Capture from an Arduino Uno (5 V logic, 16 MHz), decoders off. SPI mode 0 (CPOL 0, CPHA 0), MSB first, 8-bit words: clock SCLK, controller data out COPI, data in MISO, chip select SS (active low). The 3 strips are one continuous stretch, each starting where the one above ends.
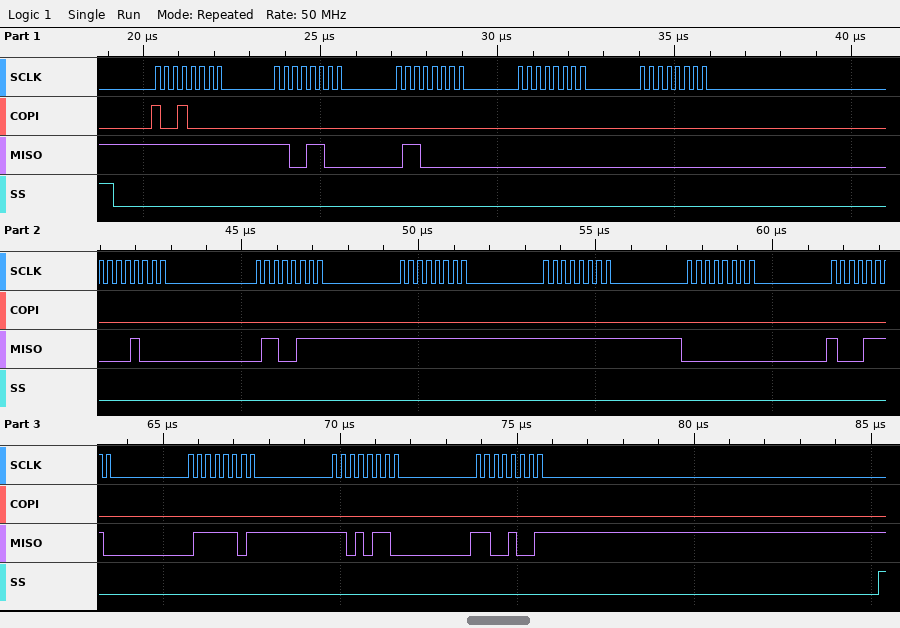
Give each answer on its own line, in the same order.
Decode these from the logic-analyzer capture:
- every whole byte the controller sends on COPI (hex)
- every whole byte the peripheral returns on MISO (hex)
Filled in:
90 00 00 00 00 00 00 00 00 00 00 00 00 00
FF CC 60 00 00 08 67 FF FF 00 8E 7D D6 C9
